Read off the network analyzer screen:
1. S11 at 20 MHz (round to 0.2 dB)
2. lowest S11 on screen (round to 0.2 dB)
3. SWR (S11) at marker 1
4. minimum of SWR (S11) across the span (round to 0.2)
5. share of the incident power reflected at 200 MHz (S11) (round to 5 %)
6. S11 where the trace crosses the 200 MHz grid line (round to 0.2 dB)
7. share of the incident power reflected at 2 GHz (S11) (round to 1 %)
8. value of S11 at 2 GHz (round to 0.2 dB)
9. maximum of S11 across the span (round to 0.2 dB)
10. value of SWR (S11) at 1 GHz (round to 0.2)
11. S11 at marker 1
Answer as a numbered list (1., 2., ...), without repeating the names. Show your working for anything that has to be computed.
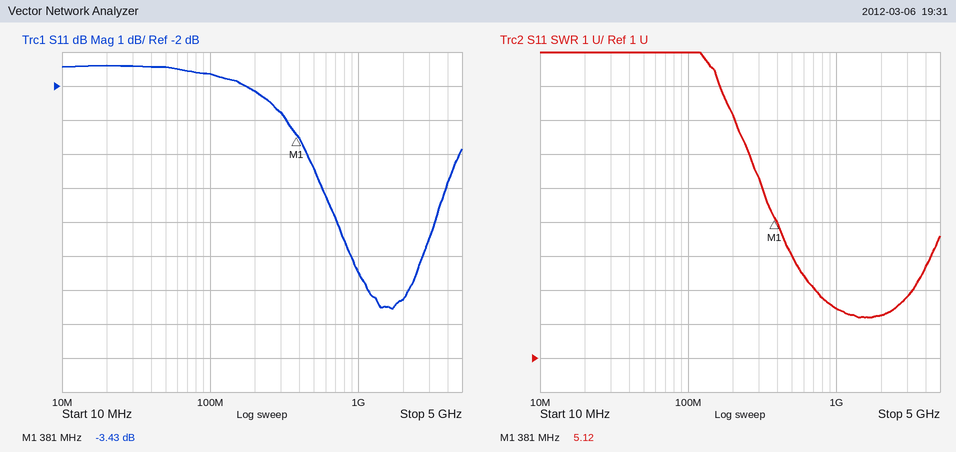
1. -1.4 dB
2. -8.6 dB
3. 5.12
4. 2.2
5. 10^(-2.2/10) ≈ 60 %
6. -2.2 dB
7. 10^(-8.2/10) ≈ 15 %
8. -8.2 dB
9. -1.4 dB
10. 2.4
11. -3.43 dB
